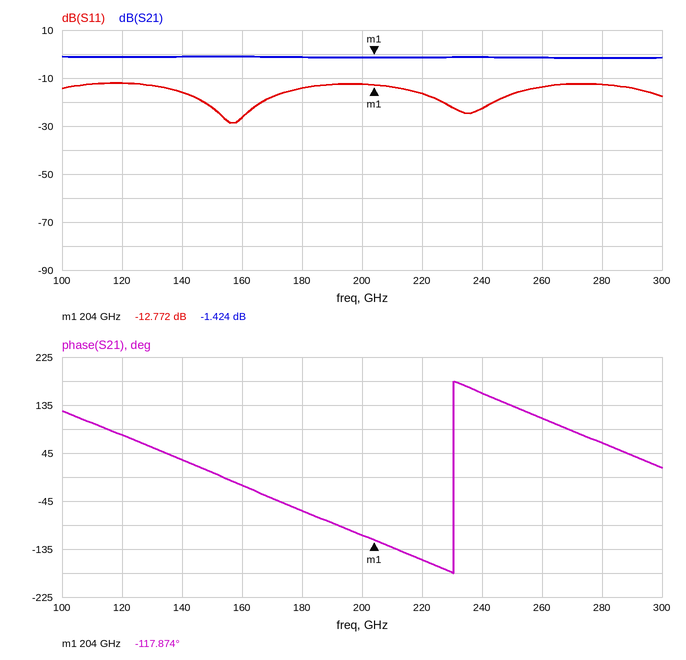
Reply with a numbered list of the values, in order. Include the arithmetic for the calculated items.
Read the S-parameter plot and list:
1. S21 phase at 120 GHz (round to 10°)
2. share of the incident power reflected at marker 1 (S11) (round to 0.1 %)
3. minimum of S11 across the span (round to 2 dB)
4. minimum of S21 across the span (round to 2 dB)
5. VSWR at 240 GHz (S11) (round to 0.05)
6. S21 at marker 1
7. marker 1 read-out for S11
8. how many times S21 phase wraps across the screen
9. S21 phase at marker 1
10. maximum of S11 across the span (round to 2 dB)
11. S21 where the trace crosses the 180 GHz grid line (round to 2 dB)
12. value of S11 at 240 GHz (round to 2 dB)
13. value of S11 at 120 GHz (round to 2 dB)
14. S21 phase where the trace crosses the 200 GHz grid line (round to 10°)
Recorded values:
1. 80°
2. 10^(-12.772/10) ≈ 5.3 %
3. -28 dB
4. -2 dB
5. |Γ| = 10^(-22/20) = 0.0794; VSWR = (1 + 0.0794)/(1 − 0.0794) ≈ 1.17, so 1.15 to the nearest 0.05
6. -1.424 dB
7. -12.772 dB
8. 1
9. -117.874°
10. -12 dB
11. -2 dB
12. -22 dB
13. -12 dB
14. -110°
